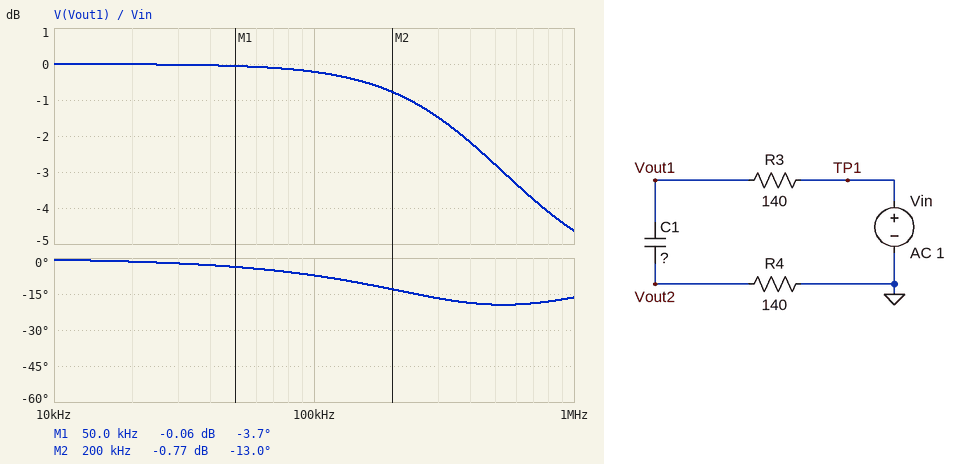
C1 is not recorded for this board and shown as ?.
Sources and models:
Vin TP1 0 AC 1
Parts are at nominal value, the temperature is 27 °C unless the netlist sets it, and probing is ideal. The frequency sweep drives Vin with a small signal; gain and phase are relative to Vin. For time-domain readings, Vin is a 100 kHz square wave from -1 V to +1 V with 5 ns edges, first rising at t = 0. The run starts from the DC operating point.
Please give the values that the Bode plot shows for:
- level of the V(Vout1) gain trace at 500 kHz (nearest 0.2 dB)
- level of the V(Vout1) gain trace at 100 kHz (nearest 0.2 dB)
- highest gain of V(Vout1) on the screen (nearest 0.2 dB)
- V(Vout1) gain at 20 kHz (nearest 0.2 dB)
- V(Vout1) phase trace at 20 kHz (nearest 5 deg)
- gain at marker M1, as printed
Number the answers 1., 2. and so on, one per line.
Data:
1. -2.8 dB
2. -0.2 dB
3. 0 dB
4. 0 dB
5. 0 deg
6. -0.06 dB
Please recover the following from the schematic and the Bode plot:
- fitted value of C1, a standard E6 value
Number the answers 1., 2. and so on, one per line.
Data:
1. 1.5 nF
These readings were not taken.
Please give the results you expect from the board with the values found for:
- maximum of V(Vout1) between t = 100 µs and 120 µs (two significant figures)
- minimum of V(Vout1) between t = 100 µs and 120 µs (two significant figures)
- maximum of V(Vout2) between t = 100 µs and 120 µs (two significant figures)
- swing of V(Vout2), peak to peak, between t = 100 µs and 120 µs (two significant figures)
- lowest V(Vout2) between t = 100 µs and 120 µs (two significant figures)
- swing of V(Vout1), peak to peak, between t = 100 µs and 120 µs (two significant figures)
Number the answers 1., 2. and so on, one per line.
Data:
1. 1.0 V
2. -1.0 V
3. 990 mV
4. 2.0 V
5. -990 mV
6. 2.0 V
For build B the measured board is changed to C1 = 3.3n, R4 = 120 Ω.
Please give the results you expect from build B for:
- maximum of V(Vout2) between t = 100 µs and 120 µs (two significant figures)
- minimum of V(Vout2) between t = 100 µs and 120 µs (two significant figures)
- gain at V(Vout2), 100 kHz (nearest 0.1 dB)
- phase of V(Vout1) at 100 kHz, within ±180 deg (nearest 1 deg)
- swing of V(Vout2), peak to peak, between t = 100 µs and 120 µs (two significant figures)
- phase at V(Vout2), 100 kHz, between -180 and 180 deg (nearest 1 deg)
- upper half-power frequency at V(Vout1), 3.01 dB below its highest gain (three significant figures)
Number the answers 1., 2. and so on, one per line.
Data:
1. 920 mV
2. -920 mV
3. -13.2 dB
4. -14 deg
5. 1.8 V
6. 62 deg
7. 245 kHz
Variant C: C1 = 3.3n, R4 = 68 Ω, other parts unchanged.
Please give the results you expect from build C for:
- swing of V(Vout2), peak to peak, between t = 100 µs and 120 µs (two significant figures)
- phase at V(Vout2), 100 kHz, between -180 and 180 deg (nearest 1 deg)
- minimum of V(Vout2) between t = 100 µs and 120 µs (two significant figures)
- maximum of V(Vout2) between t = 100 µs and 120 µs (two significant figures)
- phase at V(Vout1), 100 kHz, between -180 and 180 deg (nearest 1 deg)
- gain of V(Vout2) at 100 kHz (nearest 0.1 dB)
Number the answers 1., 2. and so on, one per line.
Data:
1. 1.3 V
2. 67 deg
3. -650 mV
4. 650 mV
5. -15 deg
6. -17.8 dB
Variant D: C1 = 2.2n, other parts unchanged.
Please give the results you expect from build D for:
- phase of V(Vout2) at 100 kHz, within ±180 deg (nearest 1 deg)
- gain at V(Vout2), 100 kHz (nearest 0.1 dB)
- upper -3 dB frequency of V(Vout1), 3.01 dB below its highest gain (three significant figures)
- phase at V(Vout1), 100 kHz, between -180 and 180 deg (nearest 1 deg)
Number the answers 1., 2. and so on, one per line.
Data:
1. 69 deg
2. -14.9 dB
3. 365 kHz
4. -10 deg
